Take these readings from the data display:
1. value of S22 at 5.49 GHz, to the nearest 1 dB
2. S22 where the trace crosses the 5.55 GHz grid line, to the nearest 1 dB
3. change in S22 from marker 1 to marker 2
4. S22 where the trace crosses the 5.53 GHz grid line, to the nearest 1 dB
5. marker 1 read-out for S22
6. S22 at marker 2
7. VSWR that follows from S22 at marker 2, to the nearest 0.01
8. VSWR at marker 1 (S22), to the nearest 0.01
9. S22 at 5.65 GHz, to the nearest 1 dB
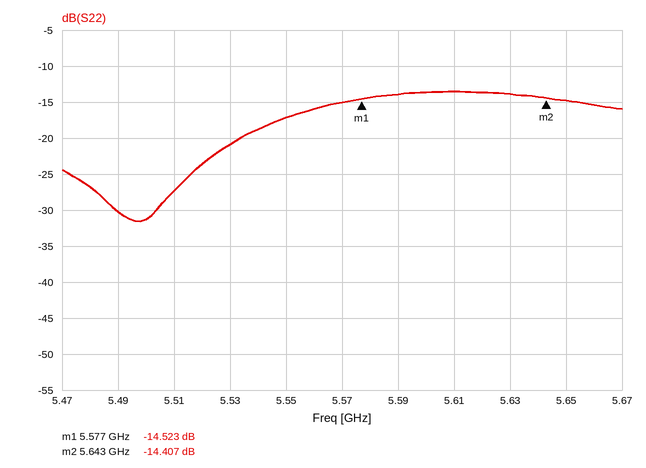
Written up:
-30 dB
-17 dB
0.116 dB
-21 dB
-14.523 dB
-14.407 dB
1.47
1.46
-15 dB
